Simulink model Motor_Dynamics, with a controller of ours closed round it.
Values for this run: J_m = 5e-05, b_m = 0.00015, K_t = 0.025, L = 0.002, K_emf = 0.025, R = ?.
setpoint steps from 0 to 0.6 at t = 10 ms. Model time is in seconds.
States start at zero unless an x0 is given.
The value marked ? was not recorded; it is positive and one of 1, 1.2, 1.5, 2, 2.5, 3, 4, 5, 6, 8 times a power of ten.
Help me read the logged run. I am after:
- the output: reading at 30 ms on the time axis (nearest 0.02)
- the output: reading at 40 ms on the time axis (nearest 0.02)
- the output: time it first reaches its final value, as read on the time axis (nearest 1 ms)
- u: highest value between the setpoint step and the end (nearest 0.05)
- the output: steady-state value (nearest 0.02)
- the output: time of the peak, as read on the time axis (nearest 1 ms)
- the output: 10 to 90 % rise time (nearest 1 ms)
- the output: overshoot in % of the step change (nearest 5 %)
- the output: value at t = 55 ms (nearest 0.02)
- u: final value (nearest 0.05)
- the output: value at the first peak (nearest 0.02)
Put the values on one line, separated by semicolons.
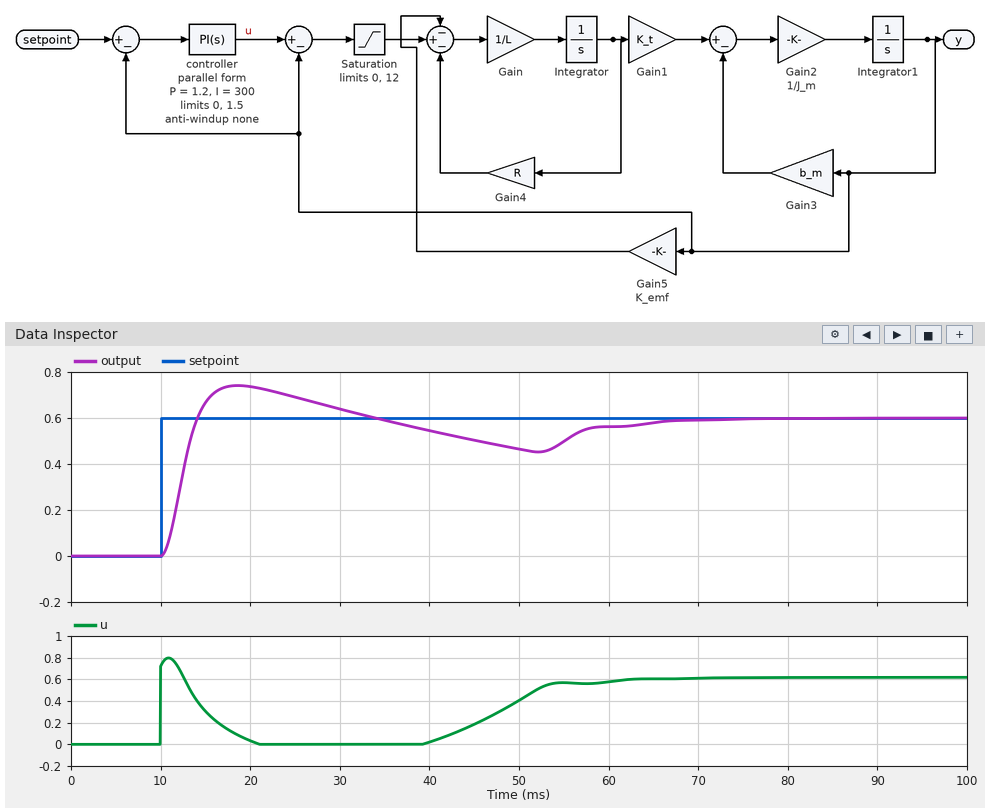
0.64; 0.54; 14 ms; 0.80; 0.60; 19 ms; 3 ms; 25 %; 0.50; 0.60; 0.74
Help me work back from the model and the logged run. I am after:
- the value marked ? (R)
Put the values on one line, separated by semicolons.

1
